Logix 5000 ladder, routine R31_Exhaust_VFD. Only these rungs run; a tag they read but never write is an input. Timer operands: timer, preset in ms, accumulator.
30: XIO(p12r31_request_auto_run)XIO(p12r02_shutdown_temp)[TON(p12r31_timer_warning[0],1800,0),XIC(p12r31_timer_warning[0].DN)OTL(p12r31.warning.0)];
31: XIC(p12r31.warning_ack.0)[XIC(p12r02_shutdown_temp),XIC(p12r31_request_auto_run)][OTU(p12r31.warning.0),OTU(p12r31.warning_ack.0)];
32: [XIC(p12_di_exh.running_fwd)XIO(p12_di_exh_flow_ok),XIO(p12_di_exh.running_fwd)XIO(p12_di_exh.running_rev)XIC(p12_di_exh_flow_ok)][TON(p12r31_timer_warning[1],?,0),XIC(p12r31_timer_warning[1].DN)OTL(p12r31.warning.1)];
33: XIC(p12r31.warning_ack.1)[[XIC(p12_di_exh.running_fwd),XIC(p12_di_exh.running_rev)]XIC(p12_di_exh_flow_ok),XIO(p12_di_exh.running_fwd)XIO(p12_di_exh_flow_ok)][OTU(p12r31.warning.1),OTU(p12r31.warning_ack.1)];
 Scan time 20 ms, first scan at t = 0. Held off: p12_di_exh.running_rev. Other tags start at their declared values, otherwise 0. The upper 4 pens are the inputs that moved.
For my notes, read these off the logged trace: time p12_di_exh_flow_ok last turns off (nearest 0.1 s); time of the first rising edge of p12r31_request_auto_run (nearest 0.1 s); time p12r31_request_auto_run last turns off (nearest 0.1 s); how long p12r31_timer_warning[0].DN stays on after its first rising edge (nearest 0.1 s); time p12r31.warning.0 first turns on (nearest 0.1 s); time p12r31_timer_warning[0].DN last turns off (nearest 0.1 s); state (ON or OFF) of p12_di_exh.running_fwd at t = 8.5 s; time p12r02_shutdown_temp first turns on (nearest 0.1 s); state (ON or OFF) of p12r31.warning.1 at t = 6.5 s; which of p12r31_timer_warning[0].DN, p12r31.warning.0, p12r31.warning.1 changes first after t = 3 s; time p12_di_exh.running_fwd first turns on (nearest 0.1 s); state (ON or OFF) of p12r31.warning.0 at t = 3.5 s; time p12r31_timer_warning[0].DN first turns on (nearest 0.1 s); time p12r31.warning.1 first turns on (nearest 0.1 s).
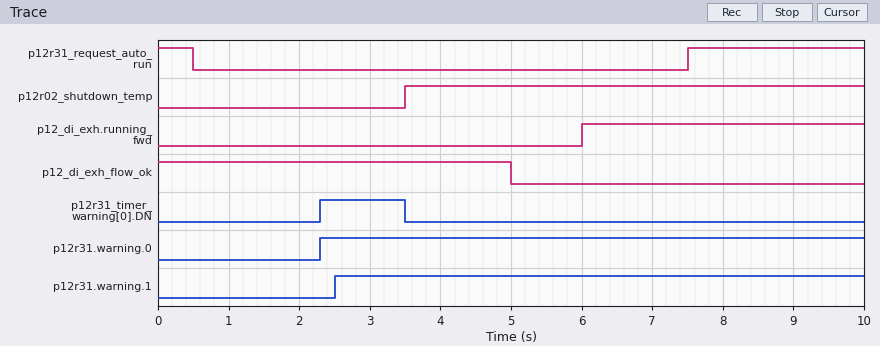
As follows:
5.0 s
7.5 s
0.5 s
1.2 s
2.3 s
3.5 s
ON
3.5 s
ON
p12r31_timer_warning[0].DN
6.0 s
ON
2.3 s
2.5 s
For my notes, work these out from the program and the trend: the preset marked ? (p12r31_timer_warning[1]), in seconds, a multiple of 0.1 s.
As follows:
2.5 s
